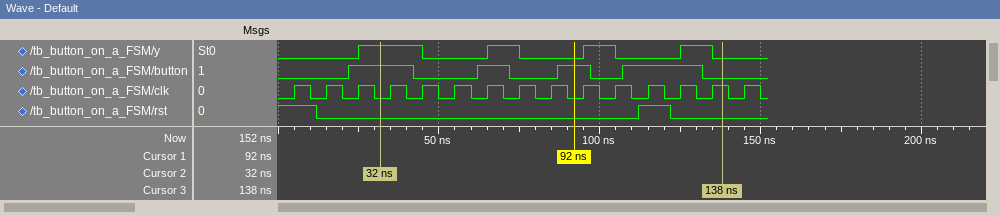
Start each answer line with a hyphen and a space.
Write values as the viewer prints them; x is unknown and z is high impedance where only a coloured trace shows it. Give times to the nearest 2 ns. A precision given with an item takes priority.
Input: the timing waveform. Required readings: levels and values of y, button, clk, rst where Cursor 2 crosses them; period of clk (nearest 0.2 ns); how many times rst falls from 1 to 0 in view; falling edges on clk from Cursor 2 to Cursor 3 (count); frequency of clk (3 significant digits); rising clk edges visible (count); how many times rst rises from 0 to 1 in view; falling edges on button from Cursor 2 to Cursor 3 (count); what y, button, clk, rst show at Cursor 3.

- y=1, button=1, clk=0, rst=0
- 10 ns
- 2
- 10
- 100 MHz
- 15
- 1
- 4
- y=0, button=0, clk=1, rst=0
